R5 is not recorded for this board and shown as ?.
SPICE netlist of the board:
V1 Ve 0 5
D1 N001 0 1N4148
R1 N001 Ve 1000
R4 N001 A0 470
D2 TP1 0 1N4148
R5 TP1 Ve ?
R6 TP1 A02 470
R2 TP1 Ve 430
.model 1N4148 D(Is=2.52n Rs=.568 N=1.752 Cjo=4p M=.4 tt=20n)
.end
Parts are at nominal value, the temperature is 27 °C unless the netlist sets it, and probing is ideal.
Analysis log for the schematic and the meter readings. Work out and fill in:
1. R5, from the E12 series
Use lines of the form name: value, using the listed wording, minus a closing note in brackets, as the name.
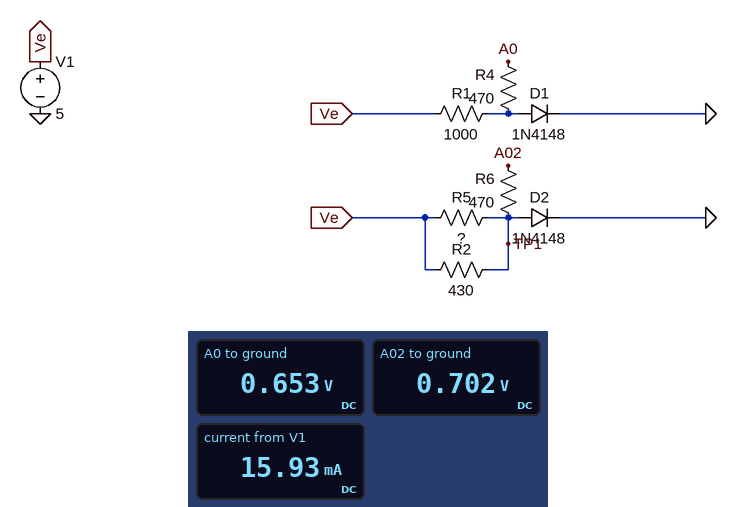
R5, from the E12 series: 2.7 kΩ
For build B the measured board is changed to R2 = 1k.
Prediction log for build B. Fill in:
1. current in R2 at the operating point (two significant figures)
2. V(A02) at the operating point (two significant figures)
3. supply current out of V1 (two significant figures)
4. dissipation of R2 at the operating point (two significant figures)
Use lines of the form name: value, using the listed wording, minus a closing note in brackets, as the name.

current in R2 at the operating point: 4.3 mA
V(A02) at the operating point: 670 mV
supply current out of V1: 10 mA
dissipation of R2 at the operating point: 19 mW
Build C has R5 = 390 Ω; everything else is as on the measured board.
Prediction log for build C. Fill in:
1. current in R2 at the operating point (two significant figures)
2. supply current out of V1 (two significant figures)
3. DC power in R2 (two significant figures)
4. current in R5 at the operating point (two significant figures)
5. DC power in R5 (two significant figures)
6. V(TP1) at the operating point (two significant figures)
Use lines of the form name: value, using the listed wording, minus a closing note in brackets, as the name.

current in R2 at the operating point: 9.9 mA
supply current out of V1: 25 mA
DC power in R2: 42 mW
current in R5 at the operating point: 11 mA
DC power in R5: 47 mW
V(TP1) at the operating point: 730 mV
